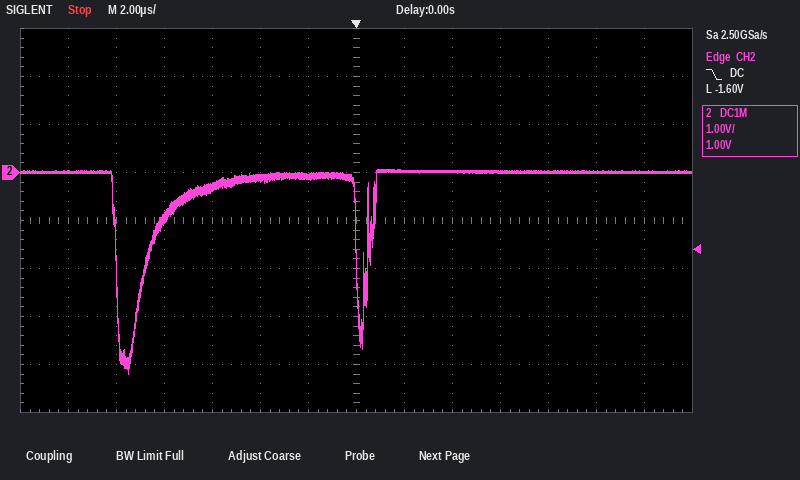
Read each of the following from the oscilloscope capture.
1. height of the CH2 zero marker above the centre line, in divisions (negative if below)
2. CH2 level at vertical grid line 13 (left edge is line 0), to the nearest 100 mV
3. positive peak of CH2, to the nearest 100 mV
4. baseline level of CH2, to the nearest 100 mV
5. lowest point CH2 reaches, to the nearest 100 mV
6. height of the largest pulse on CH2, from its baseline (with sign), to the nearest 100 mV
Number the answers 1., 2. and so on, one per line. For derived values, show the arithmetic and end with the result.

1. +1.0 div
2. 0.0 V
3. 100 mV
4. 0.0 V
5. -4.2 V
6. -4.2 V − (0.0 V) = -4.2 V
